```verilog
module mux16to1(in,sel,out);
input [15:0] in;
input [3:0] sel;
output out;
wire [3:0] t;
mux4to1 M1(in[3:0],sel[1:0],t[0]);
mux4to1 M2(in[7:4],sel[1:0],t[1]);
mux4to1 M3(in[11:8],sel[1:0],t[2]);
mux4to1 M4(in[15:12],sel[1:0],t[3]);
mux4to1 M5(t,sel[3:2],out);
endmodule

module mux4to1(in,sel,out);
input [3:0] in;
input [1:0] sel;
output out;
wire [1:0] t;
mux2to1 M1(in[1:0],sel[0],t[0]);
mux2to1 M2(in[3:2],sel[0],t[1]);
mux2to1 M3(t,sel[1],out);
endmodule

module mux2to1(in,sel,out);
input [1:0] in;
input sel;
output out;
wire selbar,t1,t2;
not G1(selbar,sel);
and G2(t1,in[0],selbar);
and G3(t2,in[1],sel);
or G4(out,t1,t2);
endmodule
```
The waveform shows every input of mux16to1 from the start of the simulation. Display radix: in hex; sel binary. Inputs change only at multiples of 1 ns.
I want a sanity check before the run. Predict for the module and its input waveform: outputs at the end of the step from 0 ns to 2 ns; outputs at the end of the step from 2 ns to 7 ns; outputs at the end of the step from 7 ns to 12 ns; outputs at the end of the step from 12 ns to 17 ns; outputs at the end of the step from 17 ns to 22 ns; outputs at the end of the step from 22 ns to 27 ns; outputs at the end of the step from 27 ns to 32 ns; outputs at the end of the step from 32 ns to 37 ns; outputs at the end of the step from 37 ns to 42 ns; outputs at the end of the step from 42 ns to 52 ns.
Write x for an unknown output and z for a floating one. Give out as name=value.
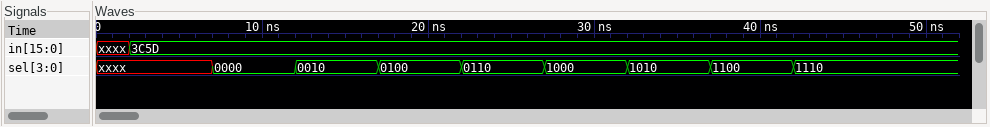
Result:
out=x
out=x
out=1
out=1
out=1
out=1
out=0
out=1
out=1
out=0
